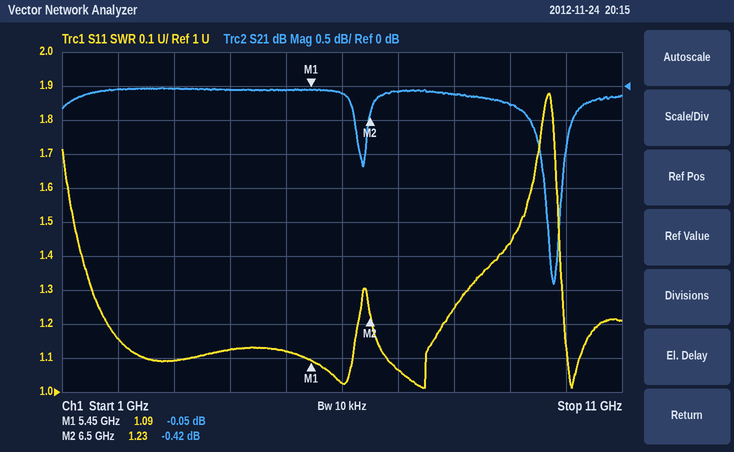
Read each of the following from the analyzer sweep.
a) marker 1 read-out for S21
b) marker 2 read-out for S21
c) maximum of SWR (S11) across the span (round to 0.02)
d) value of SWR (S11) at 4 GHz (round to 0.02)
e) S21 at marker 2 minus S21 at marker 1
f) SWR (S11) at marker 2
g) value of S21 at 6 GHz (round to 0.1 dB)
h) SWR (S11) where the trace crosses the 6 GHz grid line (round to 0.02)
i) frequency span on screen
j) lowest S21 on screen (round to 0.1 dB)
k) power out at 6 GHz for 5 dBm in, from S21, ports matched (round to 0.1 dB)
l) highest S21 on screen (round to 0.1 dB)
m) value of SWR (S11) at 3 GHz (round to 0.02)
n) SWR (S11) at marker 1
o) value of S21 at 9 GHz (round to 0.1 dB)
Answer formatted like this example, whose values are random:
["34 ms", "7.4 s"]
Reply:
["-0.05 dB", "-0.42 dB", "1.88", "1.12", "-0.37 dB", "1.23", "-0.1 dB", "1.02", "10 GHz", "-2.9 dB", "4.9 dBm", "0.0 dB", "1.10", "1.09", "-0.3 dB"]
